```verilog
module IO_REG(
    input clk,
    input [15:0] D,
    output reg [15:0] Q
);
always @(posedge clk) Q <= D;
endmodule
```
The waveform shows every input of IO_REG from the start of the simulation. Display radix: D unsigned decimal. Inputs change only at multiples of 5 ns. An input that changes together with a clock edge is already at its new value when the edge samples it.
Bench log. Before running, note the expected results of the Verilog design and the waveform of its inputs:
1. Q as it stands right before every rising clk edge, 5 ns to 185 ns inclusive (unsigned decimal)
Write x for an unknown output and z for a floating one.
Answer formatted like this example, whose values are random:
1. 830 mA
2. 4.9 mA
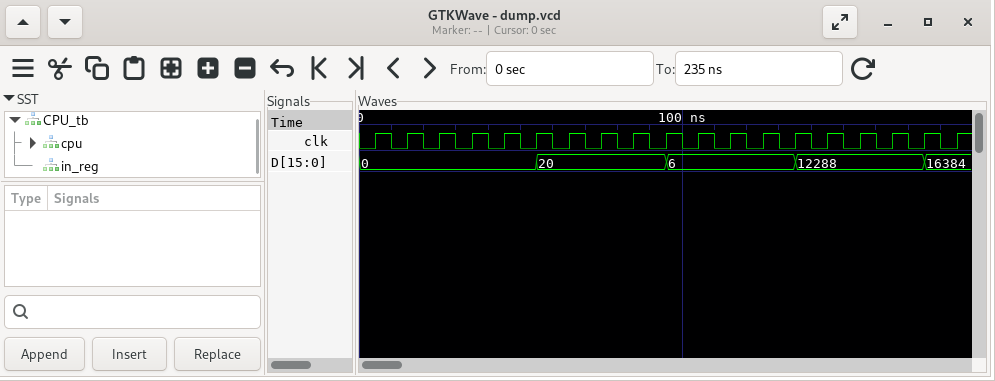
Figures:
1. x, 0, 0, 0, 0, 0, 20, 20, 20, 20, 6, 6, 6, 6, 12288, 12288, 12288, 12288, 16384
